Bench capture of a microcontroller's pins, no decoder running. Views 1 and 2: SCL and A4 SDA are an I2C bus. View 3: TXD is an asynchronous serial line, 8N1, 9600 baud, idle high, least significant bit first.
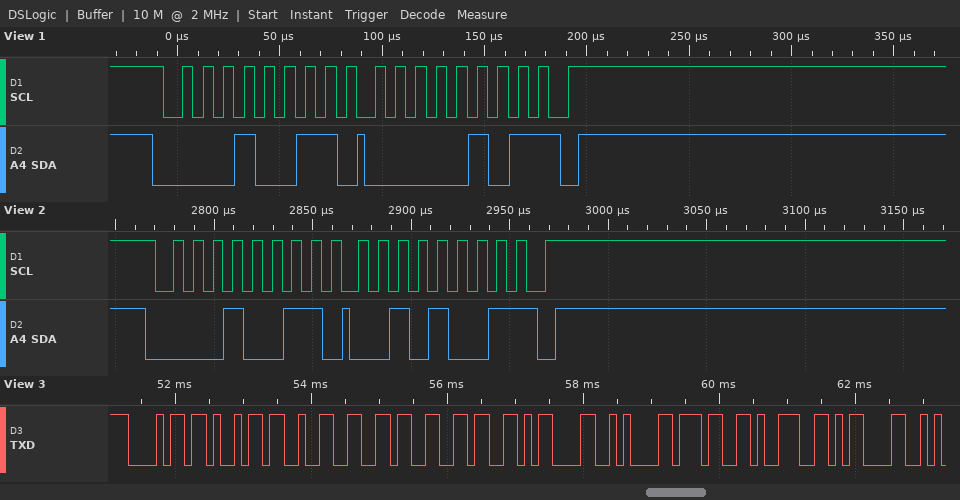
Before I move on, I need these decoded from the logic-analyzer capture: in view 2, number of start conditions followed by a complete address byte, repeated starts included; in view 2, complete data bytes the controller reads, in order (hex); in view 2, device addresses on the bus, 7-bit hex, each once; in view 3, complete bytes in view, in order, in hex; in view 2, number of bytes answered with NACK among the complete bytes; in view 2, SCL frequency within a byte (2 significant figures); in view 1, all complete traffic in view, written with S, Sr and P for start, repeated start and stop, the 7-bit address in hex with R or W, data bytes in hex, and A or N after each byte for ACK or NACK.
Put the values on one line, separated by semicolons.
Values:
1; 29; 0x09; 0x68 0x69 0x32 0x36 0x36 0x0D 0x0A 0x37 0x39 0x0D; 1; 100 kHz; S 09R A 05 N P
